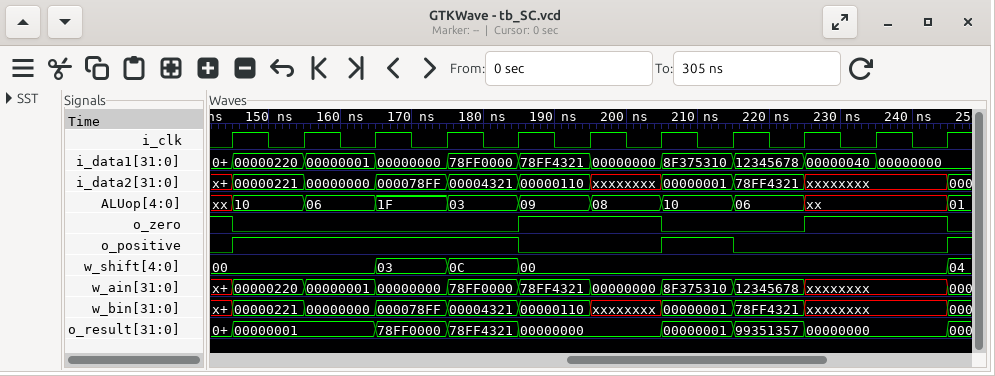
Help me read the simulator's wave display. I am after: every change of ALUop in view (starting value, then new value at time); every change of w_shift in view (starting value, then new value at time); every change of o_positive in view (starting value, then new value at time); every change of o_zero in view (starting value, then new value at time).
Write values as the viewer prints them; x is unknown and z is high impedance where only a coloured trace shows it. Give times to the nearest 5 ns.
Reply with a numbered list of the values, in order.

1. xx, 10 at 145 ns, 06 at 155 ns, 1F at 165 ns, 03 at 175 ns, 09 at 185 ns, 08 at 195 ns, 10 at 205 ns, 06 at 215 ns, xx at 225 ns, 01 at 245 ns
2. 00, 03 at 165 ns, 0C at 175 ns, 00 at 185 ns, 04 at 245 ns
3. 0, 1 at 145 ns, 0 at 185 ns, 1 at 205 ns, 0 at 215 ns, 1 at 245 ns
4. 1, 0 at 145 ns, 1 at 185 ns, 0 at 205 ns, 1 at 225 ns, 0 at 245 ns
